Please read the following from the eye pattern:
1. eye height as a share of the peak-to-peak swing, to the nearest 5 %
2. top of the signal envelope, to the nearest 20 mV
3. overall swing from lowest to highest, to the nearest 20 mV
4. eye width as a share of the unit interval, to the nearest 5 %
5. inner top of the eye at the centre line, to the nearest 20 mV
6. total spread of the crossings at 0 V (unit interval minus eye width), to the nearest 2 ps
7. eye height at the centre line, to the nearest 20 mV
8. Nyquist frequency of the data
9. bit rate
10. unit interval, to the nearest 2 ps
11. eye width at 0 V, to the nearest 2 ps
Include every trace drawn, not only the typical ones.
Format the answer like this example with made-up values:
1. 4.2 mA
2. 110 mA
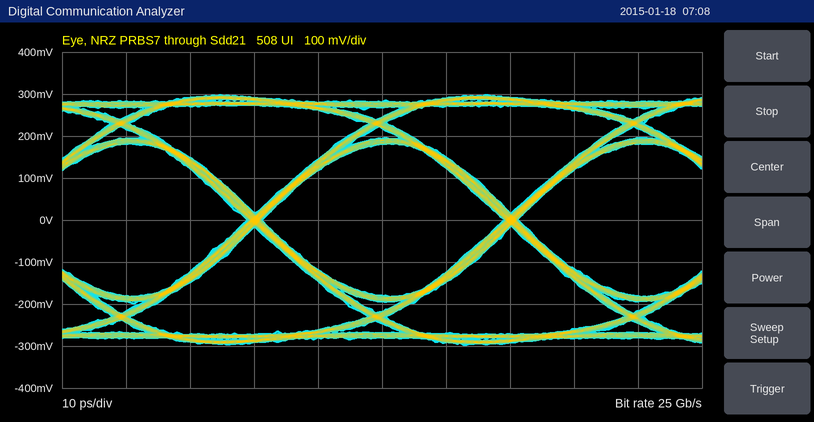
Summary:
1. 60 %
2. 300 mV
3. 600 mV
4. 95 %
5. 180 mV
6. 2 ps
7. 360 mV
8. 12.5 GHz
9. 25 Gb/s
10. 40 ps
11. 38 ps
